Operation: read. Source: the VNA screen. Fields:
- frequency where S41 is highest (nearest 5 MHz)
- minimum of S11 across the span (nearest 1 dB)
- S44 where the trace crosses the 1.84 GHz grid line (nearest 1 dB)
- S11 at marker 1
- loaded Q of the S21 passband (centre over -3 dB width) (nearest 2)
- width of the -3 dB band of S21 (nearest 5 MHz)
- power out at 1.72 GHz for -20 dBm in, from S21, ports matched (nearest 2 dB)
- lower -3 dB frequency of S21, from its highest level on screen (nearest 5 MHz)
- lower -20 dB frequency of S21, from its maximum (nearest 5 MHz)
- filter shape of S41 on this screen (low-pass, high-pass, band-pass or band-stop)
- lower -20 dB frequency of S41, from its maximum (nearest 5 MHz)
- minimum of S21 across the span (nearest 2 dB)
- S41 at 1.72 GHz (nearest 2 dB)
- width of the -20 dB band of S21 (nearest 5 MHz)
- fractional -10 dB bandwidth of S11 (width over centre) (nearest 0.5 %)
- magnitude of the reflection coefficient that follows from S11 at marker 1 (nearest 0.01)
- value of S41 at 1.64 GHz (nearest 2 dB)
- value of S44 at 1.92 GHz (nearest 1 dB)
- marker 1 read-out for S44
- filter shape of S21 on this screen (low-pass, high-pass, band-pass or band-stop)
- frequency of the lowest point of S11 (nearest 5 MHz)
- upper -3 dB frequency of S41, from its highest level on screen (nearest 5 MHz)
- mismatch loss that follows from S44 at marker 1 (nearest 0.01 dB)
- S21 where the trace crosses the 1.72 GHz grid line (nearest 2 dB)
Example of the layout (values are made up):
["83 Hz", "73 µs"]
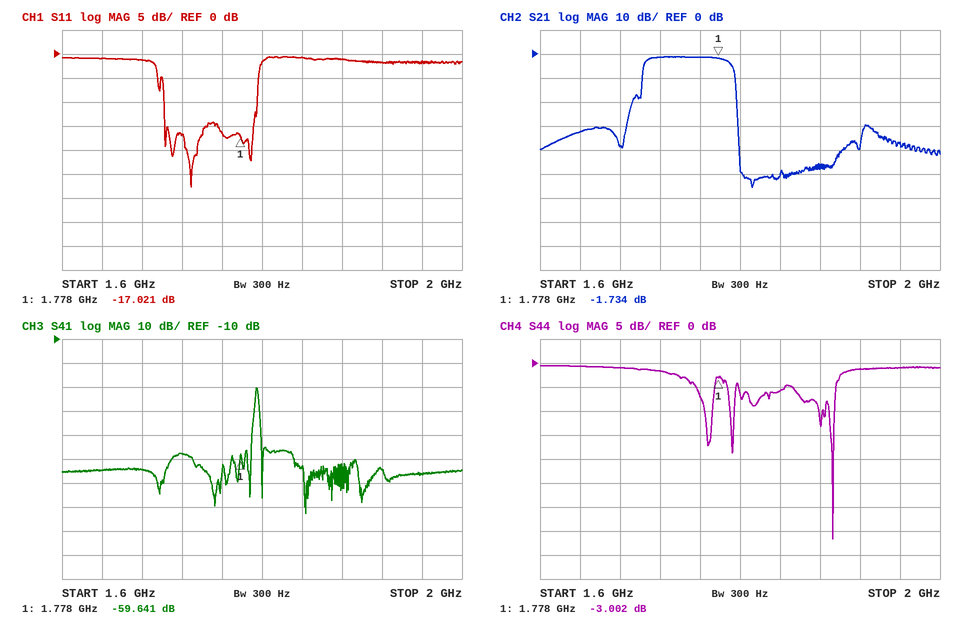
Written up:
["1.795 GHz", "-28 dB", "-6 dB", "-17.021 dB", "20", "85 MHz", "-22 dBm", "1.705 GHz", "1.690 GHz", "band-pass", "1.790 GHz", "-56 dB", "-58 dB", "105 MHz", "5.5 %", "0.14", "-64 dB", "-1 dB", "-3.002 dB", "band-pass", "1.730 GHz", "1.795 GHz", "3.02 dB", "-2 dB"]
